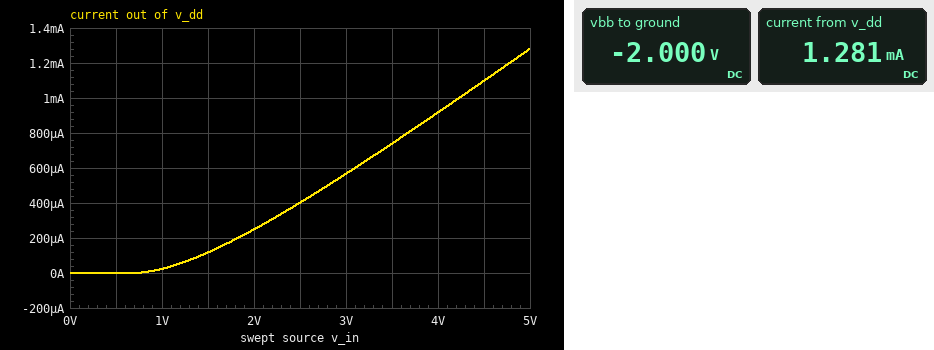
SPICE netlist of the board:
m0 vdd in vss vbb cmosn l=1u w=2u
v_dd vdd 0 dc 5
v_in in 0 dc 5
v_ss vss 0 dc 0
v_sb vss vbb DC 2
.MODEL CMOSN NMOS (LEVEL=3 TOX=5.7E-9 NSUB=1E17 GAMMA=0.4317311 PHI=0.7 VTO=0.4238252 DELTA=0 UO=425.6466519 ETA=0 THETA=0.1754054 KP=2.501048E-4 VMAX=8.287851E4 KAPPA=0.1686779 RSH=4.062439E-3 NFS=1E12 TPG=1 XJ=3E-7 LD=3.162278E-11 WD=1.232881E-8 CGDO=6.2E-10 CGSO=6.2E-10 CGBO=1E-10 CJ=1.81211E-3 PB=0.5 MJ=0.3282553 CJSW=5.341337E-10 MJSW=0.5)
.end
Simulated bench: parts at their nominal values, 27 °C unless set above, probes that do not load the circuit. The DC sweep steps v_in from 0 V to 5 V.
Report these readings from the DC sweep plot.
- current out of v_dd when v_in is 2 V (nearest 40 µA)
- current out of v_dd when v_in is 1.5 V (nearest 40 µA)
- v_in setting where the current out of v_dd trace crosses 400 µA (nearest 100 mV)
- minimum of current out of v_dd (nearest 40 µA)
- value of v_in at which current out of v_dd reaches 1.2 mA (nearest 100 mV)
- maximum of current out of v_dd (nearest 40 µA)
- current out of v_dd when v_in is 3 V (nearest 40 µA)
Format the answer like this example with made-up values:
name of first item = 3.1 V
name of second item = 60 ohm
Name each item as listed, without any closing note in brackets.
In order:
current out of v_dd when v_in is 2 V = 240 µA
current out of v_dd when v_in is 1.5 V = 120 µA
v_in setting where the current out of v_dd trace crosses 400 µA = 2.5 V
minimum of current out of v_dd = 0 A
value of v_in at which current out of v_dd reaches 1.2 mA = 4.8 V
maximum of current out of v_dd = 1.28 mA
current out of v_dd when v_in is 3 V = 560 µA
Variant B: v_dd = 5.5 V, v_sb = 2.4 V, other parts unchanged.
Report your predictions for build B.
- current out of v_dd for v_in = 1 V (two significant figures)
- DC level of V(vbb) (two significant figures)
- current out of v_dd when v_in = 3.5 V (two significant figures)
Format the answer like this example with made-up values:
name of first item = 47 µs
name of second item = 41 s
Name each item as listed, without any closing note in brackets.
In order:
current out of v_dd for v_in = 1 V = 20 µA
DC level of V(vbb) = -2.4 V
current out of v_dd when v_in = 3.5 V = 730 µA
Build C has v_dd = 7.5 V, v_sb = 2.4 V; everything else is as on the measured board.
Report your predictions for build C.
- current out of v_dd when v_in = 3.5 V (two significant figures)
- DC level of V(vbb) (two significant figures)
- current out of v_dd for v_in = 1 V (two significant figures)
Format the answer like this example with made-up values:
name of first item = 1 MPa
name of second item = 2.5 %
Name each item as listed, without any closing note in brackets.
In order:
current out of v_dd when v_in = 3.5 V = 750 µA
DC level of V(vbb) = -2.4 V
current out of v_dd for v_in = 1 V = 20 µA
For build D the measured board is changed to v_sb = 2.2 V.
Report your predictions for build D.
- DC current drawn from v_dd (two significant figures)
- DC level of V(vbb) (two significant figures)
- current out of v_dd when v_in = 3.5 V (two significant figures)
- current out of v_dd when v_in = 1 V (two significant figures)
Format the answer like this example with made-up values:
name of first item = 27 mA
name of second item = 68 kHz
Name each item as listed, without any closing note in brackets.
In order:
DC current drawn from v_dd = 1.3 mA
DC level of V(vbb) = -2.2 V
current out of v_dd when v_in = 3.5 V = 730 µA
current out of v_dd when v_in = 1 V = 22 µA
